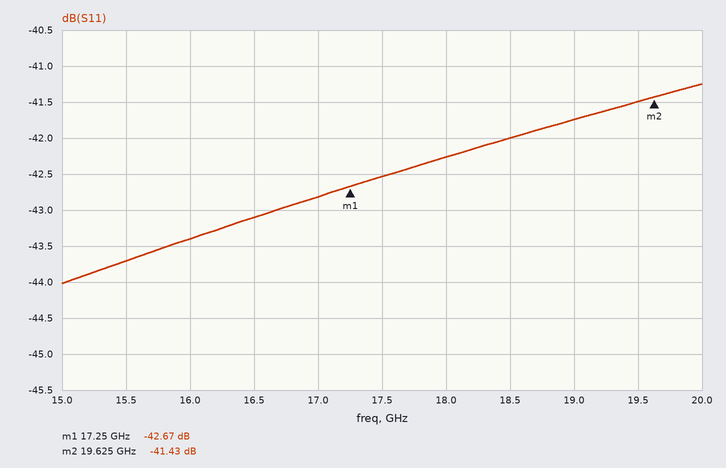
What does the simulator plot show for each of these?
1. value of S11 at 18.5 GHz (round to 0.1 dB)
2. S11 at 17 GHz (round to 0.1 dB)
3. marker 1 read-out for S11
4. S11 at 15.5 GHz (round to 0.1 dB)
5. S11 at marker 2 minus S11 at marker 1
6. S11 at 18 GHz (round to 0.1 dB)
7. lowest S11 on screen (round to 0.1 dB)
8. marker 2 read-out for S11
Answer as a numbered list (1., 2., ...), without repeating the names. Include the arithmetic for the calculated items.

1. -42.0 dB
2. -42.8 dB
3. -42.67 dB
4. -43.7 dB
5. -41.43 − (-42.67) = 1.24 dB
6. -42.3 dB
7. -44.0 dB
8. -41.43 dB
